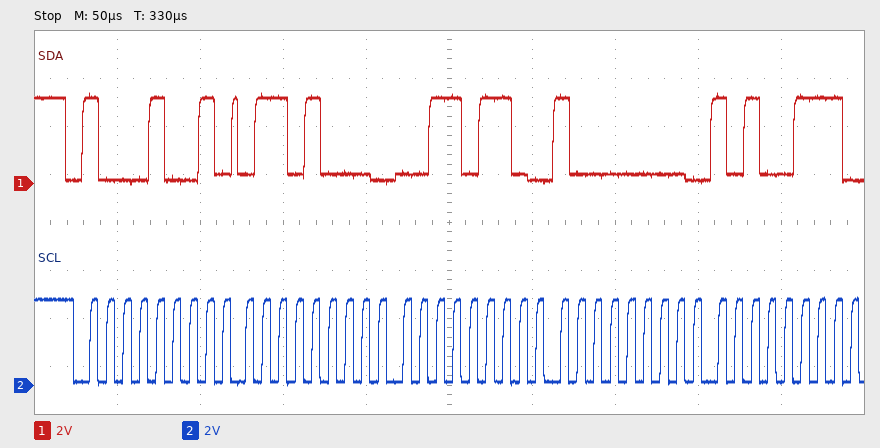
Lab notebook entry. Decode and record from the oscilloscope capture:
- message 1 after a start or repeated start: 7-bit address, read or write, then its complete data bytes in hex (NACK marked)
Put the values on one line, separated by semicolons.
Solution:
0x44 read: 68 36 80 A7
